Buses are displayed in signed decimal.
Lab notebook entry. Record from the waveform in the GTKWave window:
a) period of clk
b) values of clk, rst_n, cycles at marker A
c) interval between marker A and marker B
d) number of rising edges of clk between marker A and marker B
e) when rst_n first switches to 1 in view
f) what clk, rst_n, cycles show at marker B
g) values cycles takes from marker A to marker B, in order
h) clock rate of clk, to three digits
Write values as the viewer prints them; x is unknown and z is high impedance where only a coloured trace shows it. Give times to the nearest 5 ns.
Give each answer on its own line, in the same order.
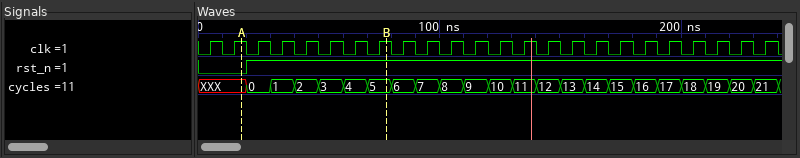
10 ns
clk=1, rst_n=0, cycles=XXX
60 ns
6
20 ns
clk=1, rst_n=1, cycles=5
XXX, 0, 1, 2, 3, 4, 5
100 MHz
